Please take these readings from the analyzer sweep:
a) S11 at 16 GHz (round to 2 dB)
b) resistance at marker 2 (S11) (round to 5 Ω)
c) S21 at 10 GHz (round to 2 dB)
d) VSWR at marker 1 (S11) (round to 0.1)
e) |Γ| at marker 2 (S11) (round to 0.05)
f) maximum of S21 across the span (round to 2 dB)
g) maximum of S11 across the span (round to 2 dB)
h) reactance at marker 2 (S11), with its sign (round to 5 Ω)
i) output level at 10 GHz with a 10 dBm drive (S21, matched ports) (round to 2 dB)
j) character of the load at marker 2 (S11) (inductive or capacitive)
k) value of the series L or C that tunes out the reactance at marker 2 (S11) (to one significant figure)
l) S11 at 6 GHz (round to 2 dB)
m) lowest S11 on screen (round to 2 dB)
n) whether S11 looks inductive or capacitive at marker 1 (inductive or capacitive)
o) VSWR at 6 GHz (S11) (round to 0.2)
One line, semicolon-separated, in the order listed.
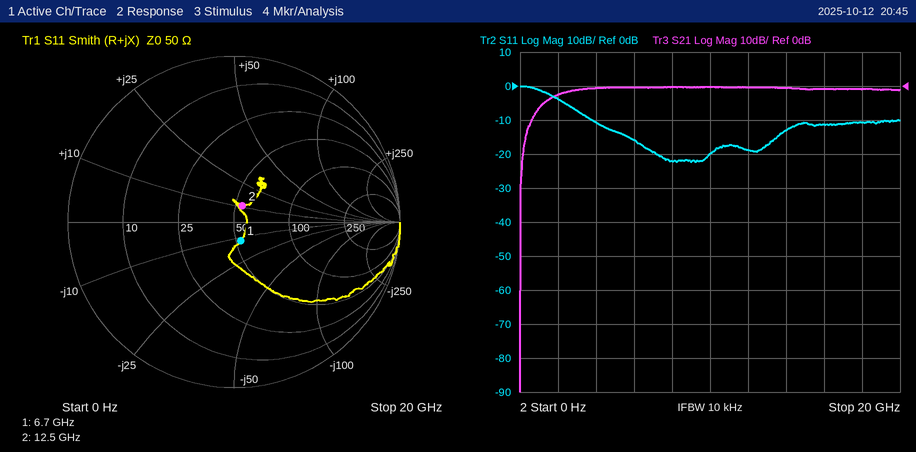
-12 dB; 55 Ω; 0 dB; 1.3; 0.10; 0 dB; 0 dB; +10 Ω; 10 dBm; inductive; 1 pF; -16 dB; -22 dB; capacitive; 1.4
